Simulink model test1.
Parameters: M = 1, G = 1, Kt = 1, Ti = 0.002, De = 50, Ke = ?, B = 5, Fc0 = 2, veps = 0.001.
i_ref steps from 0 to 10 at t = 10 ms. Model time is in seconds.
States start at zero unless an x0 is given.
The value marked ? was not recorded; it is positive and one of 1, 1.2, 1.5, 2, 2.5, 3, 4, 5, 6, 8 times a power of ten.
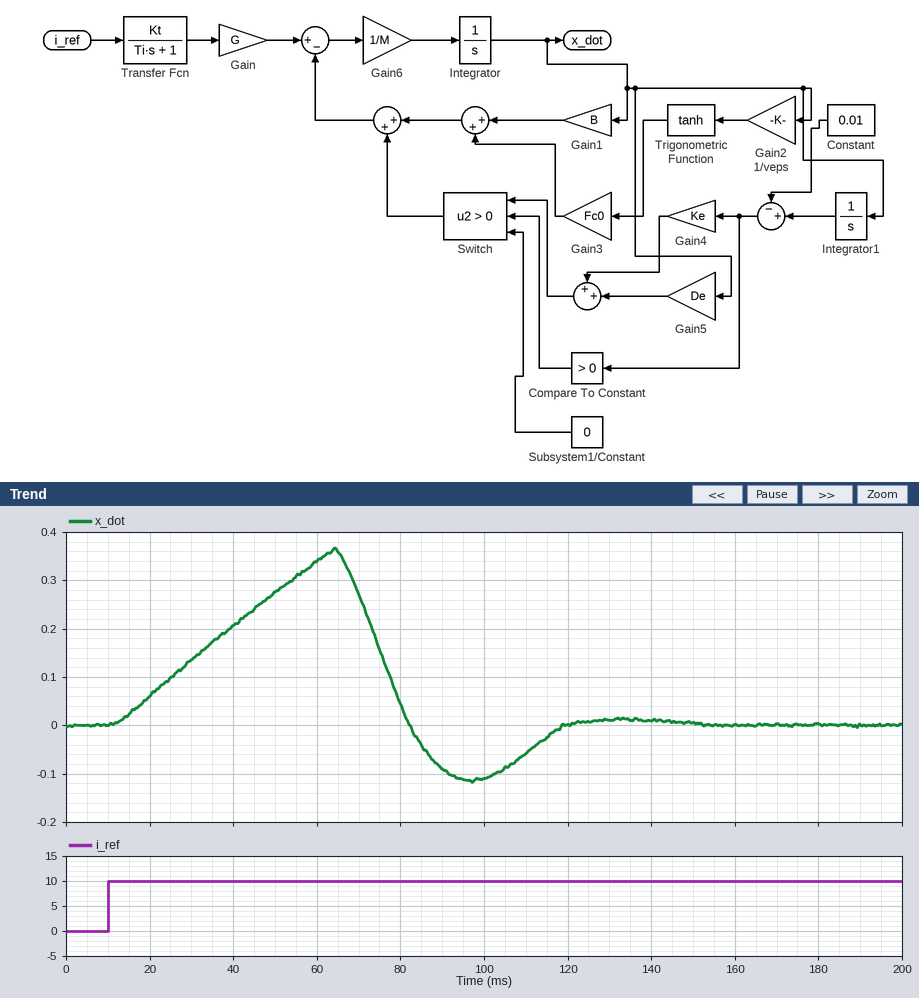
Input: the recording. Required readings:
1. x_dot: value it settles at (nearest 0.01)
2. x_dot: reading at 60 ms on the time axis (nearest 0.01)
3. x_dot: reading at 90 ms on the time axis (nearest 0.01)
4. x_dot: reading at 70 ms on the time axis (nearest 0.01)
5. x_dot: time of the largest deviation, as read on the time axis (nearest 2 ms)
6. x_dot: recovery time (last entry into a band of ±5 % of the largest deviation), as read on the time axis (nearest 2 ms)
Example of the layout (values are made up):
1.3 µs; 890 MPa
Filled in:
0.00; 0.34; -0.09; 0.27; 64 ms; 116 ms
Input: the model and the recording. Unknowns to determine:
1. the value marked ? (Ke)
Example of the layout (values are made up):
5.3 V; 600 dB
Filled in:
8000
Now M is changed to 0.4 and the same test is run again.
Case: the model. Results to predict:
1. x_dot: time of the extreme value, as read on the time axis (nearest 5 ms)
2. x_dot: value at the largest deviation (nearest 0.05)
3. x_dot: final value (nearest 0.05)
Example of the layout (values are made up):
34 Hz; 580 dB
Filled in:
45 ms; 0.55; 0.00
